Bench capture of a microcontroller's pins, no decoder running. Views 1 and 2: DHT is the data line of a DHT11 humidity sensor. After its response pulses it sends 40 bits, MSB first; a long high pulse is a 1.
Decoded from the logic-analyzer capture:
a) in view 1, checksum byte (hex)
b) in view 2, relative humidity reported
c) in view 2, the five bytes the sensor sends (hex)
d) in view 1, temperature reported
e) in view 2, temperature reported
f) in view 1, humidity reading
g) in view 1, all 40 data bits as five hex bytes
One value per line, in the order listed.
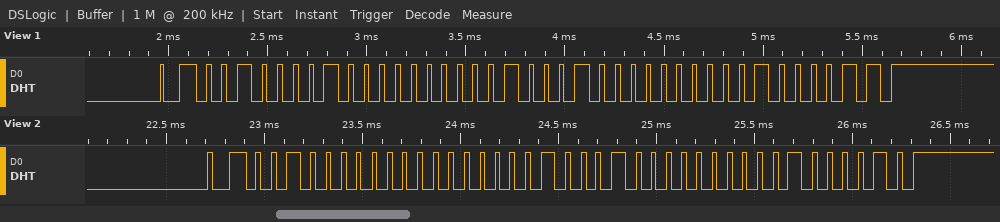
0x43
32 %
20 00 22 00 42
34.0 °C
34.0 °C
33 %
21 00 22 00 43
